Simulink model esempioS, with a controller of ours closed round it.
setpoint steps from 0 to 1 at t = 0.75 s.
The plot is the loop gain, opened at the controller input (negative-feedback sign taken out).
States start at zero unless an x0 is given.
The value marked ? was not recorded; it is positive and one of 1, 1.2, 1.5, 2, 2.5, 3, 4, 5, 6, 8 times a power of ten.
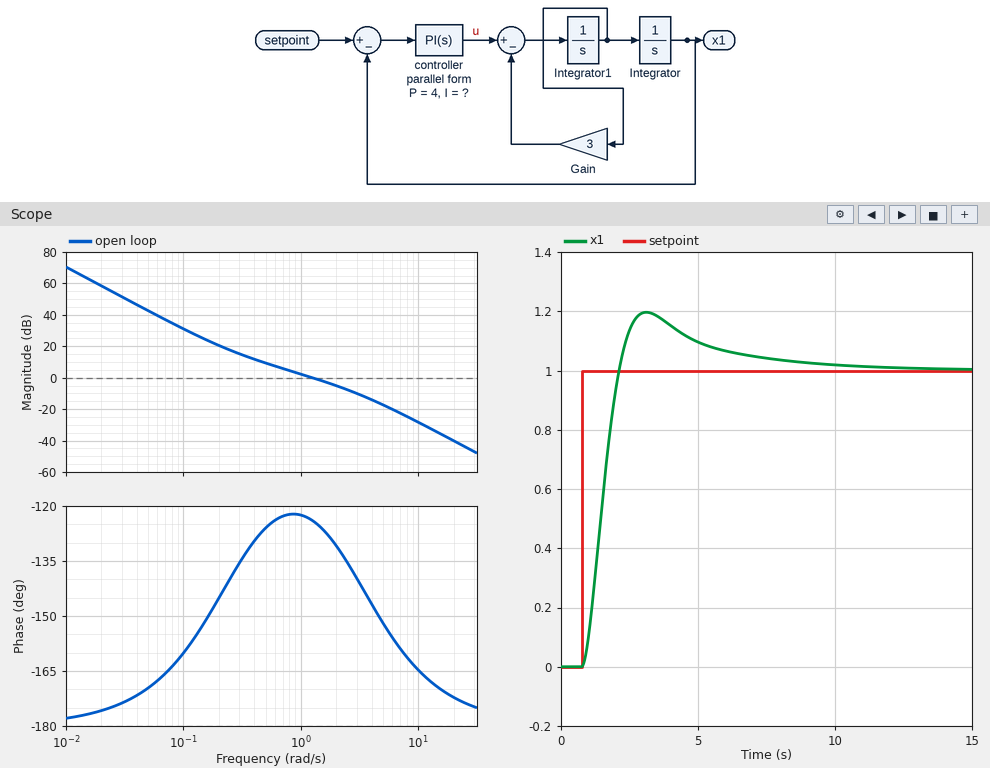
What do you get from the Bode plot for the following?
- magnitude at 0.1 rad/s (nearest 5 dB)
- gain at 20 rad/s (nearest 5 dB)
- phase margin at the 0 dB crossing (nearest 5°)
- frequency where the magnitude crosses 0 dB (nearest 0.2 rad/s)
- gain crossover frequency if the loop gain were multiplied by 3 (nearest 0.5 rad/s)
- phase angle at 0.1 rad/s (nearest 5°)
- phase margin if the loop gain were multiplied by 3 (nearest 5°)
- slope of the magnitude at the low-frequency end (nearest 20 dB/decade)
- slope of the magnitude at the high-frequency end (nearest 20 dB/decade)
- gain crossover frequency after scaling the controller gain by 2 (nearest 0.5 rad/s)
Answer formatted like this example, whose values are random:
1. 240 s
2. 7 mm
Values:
1. 30 dB
2. -40 dB
3. 55°
4. 1.2 rad/s
5. 3.0 rad/s
6. -160°
7. 40°
8. -40 dB/decade
9. -40 dB/decade
10. 2.0 rad/s
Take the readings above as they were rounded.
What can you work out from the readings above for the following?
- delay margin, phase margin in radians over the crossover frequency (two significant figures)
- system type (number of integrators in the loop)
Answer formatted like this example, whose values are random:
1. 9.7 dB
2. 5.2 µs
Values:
1. 0.80 s
2. 2
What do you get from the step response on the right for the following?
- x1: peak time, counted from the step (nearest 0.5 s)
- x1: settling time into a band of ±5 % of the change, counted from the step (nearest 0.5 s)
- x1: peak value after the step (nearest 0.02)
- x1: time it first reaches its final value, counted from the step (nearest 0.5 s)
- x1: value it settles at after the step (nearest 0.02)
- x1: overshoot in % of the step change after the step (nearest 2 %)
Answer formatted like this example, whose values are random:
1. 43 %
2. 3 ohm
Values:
1. 2.5 s
2. 6.0 s
3. 1.20
4. 1.5 s
5. 1.00
6. 20 %
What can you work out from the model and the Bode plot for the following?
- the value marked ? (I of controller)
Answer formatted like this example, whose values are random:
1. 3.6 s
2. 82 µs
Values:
1. 1
